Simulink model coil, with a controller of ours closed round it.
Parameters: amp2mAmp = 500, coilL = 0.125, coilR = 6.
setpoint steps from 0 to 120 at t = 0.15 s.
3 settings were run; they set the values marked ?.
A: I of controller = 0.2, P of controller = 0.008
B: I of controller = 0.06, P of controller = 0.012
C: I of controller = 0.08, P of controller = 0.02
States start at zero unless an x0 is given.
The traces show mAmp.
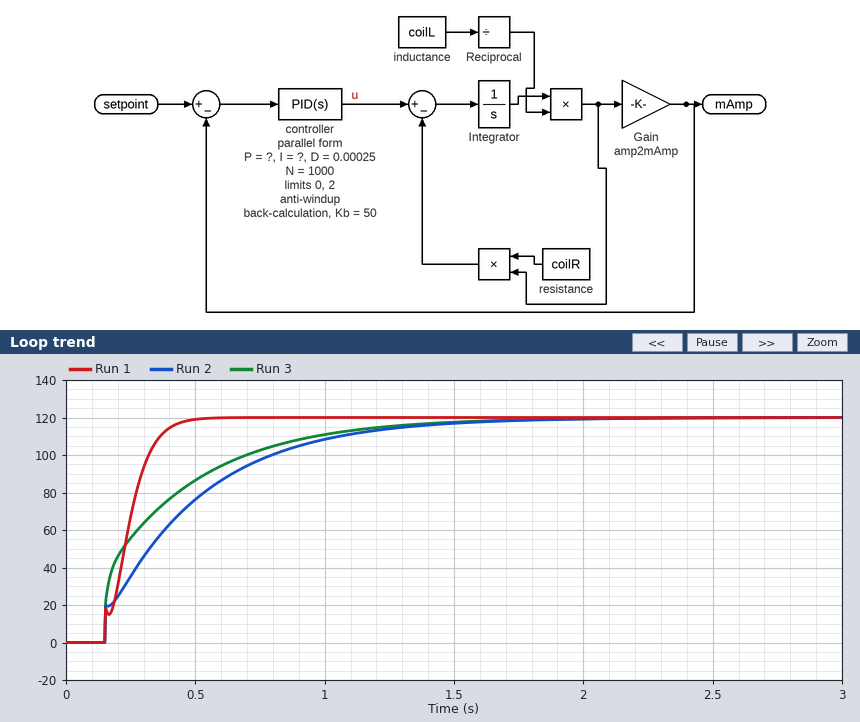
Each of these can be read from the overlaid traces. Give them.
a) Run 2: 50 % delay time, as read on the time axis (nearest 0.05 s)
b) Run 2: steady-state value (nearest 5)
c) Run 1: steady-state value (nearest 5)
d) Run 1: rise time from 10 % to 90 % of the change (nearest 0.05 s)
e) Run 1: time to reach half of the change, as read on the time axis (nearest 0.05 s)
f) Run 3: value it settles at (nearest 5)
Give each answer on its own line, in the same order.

0.40 s
120
120
0.20 s
0.25 s
120
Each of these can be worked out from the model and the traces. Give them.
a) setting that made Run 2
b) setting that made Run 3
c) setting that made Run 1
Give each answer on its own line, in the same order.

B
C
A
